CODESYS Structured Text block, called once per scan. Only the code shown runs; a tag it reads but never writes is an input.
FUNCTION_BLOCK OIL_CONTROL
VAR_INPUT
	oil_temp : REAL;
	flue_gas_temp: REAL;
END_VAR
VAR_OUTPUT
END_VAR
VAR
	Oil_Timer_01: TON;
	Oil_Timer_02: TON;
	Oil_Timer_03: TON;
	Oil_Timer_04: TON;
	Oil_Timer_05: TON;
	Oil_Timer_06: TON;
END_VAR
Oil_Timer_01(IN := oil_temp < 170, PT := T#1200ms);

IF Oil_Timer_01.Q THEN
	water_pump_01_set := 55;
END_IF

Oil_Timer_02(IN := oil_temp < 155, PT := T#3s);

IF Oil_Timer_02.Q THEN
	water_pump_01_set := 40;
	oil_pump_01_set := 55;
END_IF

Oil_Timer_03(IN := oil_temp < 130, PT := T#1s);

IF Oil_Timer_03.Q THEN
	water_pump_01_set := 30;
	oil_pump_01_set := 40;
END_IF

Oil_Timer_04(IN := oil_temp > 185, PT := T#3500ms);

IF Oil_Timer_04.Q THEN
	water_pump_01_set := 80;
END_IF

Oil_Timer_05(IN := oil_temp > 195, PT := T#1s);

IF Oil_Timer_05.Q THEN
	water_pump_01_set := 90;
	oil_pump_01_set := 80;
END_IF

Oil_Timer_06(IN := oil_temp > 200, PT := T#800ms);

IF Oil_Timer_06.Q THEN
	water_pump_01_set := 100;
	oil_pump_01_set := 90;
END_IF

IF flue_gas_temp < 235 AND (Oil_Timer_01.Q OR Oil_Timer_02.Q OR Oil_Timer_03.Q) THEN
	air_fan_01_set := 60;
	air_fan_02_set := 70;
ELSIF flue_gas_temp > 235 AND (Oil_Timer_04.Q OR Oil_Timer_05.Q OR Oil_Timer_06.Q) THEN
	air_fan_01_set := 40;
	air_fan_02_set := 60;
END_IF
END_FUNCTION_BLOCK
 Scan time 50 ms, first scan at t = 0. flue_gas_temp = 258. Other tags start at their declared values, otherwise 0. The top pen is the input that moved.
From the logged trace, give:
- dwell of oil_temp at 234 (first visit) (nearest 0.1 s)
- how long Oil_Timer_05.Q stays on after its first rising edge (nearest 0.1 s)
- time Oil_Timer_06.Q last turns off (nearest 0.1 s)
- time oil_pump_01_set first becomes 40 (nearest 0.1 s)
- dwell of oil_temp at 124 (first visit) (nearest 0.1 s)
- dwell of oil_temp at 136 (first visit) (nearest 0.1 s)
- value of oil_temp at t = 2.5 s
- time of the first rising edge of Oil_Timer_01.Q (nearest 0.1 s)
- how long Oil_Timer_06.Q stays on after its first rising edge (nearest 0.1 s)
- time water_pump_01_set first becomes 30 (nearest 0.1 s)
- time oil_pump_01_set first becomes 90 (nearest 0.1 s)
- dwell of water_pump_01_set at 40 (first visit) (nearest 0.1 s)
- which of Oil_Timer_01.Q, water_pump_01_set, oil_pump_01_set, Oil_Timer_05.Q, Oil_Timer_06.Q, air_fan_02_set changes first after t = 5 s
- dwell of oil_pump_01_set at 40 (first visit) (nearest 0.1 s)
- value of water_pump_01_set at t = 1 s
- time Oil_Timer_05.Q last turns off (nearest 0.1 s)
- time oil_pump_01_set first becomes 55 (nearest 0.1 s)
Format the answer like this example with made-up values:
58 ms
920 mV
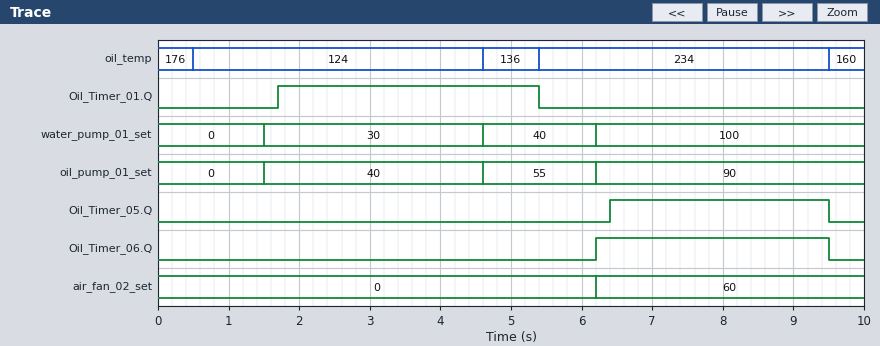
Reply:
4.1 s
3.1 s
9.5 s
1.5 s
4.1 s
0.8 s
124
1.7 s
3.3 s
1.5 s
6.2 s
1.6 s
Oil_Timer_01.Q
3.1 s
0
9.5 s
4.6 s
